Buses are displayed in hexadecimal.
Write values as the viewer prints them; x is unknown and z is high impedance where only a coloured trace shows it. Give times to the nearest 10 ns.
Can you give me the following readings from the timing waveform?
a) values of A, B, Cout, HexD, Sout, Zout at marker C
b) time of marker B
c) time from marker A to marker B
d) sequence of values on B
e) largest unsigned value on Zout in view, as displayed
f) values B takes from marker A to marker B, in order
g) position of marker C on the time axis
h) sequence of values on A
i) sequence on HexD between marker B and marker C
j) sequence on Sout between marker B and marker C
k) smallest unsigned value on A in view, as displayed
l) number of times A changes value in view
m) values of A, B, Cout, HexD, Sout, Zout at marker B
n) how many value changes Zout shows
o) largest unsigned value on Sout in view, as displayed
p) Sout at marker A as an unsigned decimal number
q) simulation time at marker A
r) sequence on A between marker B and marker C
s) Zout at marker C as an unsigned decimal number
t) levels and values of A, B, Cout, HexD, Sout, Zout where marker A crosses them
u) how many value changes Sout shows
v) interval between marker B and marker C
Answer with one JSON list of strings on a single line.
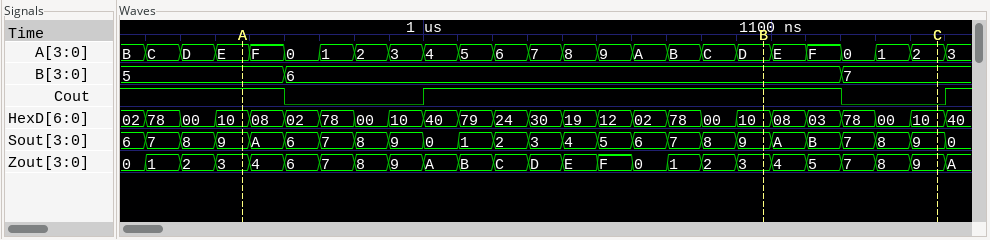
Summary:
["A=2, B=7, Cout=0, HexD=10, Sout=9, Zout=9", "1100 ns", "150 ns", "5, 6, 7", "F", "5, 6", "1150 ns", "B, C, D, E, F, 0, 1, 2, 3, 4, 5, 6, 7, 8, 9, A, B, C, D, E, F, 0, 1, 2, 3", "10, 08, 03, 78, 00, 10", "9, A, B, 7, 8, 9", "0", "24", "A=D, B=6, Cout=1, HexD=10, Sout=9, Zout=3", "24", "B", "9", "950 ns", "D, E, F, 0, 1, 2", "9", "A=E, B=5, Cout=1, HexD=10, Sout=9, Zout=3", "24", "50 ns"]
